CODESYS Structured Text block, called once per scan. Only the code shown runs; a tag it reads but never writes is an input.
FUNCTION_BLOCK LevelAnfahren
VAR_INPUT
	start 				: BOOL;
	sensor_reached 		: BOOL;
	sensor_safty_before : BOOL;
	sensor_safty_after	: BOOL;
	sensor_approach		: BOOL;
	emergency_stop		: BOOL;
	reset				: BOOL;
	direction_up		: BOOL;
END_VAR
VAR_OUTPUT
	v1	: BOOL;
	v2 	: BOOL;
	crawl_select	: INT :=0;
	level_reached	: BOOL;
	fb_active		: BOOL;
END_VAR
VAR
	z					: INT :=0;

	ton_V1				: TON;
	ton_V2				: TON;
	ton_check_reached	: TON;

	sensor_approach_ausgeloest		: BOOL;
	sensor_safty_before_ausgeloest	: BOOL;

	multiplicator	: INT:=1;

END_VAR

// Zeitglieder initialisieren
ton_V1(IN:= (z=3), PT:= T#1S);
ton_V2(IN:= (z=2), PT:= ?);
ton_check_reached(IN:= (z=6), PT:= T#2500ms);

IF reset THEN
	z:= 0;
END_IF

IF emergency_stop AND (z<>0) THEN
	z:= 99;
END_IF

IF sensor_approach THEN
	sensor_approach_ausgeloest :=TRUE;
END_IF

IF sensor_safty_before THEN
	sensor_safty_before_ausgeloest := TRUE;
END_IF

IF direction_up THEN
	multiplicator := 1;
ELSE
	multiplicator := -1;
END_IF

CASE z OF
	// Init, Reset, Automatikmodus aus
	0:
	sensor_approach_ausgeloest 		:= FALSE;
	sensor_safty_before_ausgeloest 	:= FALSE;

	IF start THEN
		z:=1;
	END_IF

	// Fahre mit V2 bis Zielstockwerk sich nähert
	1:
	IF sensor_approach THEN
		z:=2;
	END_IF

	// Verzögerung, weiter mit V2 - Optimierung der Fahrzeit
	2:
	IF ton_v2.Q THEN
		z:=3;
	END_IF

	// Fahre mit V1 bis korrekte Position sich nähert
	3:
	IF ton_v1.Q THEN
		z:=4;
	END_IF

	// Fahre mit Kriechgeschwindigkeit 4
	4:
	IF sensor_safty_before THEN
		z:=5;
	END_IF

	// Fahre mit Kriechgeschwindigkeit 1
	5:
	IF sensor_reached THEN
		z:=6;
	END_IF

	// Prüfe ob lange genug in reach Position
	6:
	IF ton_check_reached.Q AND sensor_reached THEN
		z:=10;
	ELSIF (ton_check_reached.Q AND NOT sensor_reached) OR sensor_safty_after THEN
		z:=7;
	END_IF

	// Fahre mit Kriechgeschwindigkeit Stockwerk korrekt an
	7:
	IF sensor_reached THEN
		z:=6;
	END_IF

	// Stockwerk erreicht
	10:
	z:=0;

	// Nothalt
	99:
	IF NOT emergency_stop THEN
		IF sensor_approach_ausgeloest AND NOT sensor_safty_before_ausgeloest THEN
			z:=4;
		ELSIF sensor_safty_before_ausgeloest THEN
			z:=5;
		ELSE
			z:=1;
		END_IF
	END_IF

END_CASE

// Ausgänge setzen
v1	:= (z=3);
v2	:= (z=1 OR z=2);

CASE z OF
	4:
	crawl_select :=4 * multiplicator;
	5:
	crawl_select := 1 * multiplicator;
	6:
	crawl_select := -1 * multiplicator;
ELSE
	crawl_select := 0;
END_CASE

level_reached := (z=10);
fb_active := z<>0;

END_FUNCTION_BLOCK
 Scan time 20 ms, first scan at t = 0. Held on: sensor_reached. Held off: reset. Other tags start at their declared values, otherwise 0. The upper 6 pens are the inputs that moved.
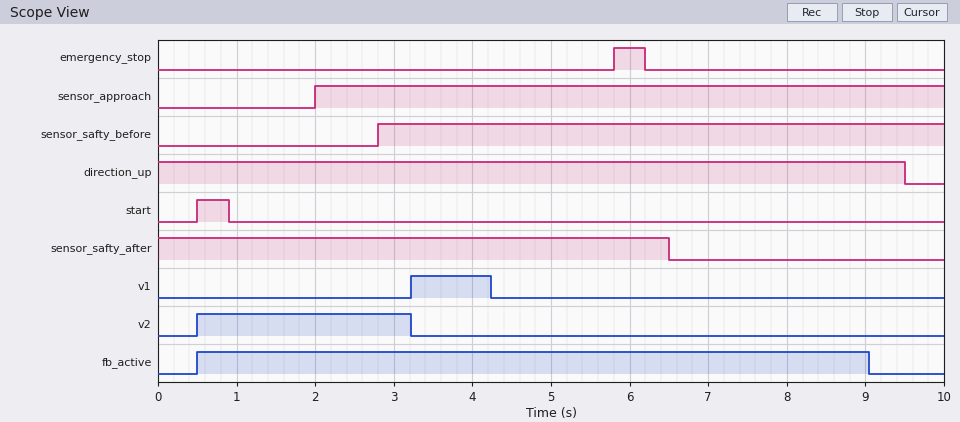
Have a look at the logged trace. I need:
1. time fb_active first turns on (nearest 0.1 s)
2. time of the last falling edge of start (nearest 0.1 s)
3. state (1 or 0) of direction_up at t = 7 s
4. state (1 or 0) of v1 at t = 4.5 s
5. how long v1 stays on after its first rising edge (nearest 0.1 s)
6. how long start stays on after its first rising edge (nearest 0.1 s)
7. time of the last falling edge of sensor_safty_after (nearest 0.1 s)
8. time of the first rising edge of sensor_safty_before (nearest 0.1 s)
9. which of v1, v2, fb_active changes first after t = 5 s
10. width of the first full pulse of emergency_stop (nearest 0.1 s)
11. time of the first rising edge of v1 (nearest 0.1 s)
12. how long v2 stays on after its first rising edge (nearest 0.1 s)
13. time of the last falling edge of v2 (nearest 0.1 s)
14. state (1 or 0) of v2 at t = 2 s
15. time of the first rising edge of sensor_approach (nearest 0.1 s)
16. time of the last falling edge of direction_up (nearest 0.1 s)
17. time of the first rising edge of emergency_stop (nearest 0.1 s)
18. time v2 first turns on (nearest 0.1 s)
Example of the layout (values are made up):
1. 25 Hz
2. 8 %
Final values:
1. 0.5 s
2. 0.9 s
3. 1
4. 0
5. 1.0 s
6. 0.4 s
7. 6.5 s
8. 2.8 s
9. fb_active
10. 0.4 s
11. 3.2 s
12. 2.7 s
13. 3.2 s
14. 1
15. 2.0 s
16. 9.5 s
17. 5.8 s
18. 0.5 s
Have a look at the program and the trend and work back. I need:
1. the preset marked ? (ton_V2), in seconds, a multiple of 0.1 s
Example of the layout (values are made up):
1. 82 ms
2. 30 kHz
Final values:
1. 1.2 s
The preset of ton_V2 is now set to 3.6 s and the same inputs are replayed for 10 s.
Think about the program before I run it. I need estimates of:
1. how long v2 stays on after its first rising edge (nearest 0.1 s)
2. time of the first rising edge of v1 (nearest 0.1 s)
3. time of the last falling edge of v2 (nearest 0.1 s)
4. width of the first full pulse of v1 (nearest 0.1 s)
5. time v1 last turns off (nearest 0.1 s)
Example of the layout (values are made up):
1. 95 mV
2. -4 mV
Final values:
1. 5.1 s
2. 5.6 s
3. 5.6 s
4. 0.2 s
5. 5.8 s
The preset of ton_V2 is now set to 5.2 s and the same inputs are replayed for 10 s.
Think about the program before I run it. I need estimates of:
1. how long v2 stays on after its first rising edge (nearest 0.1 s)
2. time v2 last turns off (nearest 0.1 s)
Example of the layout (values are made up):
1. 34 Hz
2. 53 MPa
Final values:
1. 5.3 s
2. 5.8 s
